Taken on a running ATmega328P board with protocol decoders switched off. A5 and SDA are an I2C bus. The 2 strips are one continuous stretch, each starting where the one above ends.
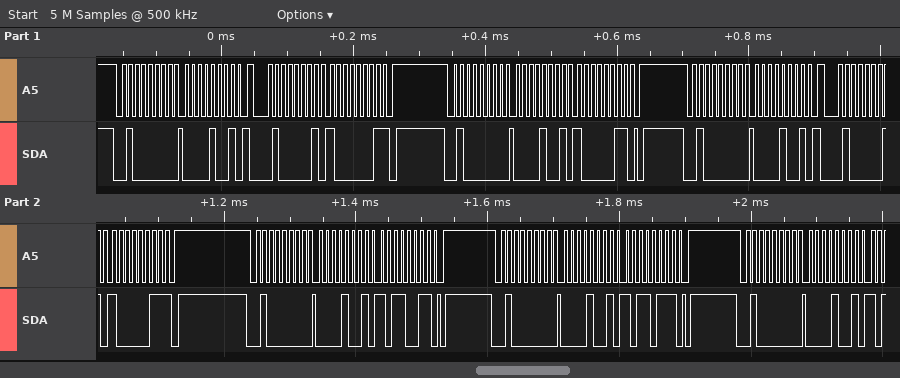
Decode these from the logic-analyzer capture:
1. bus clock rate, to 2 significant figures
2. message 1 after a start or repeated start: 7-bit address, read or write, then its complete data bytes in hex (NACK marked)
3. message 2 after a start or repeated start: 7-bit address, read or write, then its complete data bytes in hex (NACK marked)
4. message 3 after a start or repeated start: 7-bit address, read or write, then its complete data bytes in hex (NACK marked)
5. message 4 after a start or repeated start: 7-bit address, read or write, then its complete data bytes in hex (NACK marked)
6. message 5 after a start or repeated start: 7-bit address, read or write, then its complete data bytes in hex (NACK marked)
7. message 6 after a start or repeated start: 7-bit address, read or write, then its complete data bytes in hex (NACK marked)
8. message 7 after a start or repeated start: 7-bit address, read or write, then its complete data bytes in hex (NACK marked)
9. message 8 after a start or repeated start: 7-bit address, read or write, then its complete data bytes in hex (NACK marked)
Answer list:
100 kHz
0x20 write: 09
0x20 read: 81 NACK
0x20 write: 09 83
0x20 write: 09
0x20 read: 83 NACK
0x20 write: 09 B3
0x20 write: 09 B7
0x20 write: 09
